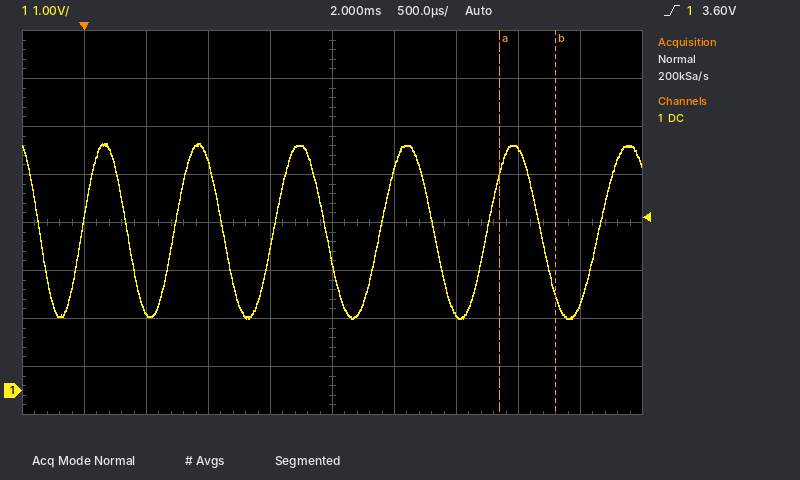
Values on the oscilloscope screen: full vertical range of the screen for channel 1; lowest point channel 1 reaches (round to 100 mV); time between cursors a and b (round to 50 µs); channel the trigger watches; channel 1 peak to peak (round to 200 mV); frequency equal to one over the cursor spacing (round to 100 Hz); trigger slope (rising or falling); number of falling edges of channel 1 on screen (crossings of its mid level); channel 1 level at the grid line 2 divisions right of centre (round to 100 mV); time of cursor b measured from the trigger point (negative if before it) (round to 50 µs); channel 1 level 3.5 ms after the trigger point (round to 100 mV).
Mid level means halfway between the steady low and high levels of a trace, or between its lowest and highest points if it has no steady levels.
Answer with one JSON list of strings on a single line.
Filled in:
["8 V", "1.5 V", "450 µs", "channel 1", "3.6 V", "2.2 kHz", "rising", "6", "1.6 V", "+3.80 ms", "5.0 V"]
